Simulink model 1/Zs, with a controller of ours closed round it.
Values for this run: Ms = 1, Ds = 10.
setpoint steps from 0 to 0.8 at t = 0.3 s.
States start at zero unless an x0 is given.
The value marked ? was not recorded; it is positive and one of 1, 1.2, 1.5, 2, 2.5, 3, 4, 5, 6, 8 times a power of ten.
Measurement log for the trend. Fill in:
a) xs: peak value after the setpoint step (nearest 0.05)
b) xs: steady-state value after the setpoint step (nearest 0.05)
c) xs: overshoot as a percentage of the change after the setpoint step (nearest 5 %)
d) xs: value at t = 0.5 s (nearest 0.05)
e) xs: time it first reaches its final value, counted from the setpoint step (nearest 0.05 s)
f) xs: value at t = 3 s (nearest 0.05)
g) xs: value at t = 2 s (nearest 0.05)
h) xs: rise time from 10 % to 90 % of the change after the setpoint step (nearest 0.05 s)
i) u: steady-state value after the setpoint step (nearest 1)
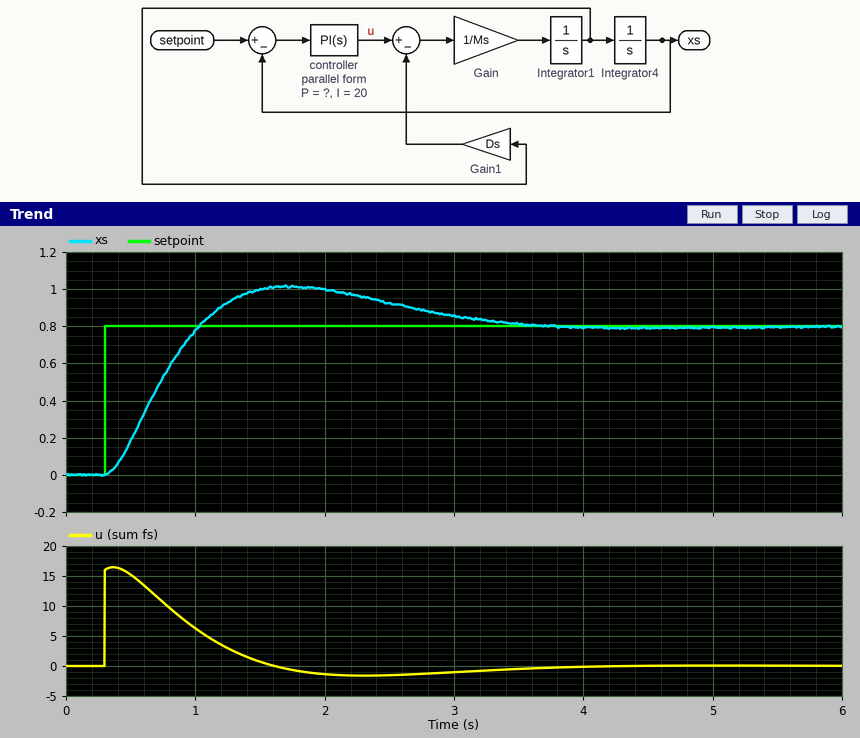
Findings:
1.00
0.80
25 %
0.20
0.75 s
0.85
1.00
0.50 s
0
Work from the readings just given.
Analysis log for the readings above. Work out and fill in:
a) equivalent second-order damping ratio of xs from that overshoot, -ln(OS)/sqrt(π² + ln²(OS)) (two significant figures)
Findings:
0.40
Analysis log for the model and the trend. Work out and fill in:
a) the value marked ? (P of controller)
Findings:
20
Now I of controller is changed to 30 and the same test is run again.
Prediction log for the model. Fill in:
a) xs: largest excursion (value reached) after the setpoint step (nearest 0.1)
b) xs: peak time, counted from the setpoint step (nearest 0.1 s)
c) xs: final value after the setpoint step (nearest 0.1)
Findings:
1.1
1.3 s
0.8
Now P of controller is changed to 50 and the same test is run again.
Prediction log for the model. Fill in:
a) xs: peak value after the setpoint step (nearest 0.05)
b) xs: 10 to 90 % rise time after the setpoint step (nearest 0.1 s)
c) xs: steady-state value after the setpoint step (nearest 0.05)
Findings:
0.90
0.3 s
0.80
